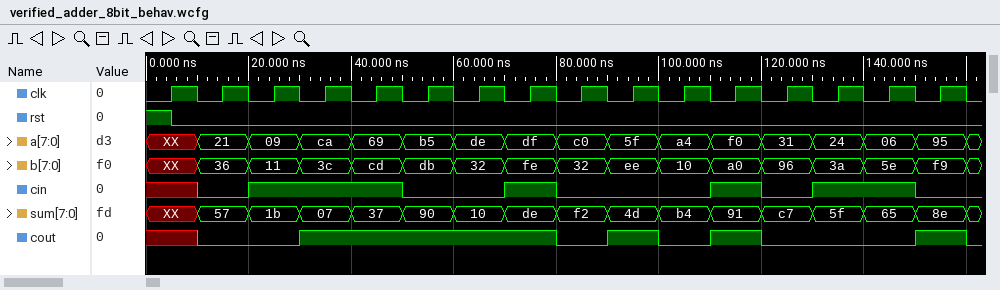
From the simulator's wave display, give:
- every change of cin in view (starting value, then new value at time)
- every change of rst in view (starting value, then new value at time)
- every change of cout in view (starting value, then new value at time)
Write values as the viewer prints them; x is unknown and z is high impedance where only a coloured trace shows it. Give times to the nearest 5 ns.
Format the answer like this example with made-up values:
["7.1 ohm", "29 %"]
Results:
["x, 0 at 10 ns, 1 at 20 ns, 0 at 50 ns, 1 at 70 ns, 0 at 80 ns, 1 at 110 ns, 0 at 120 ns, 1 at 130 ns, 0 at 150 ns", "1, 0 at 5 ns", "x, 0 at 10 ns, 1 at 30 ns, 0 at 80 ns, 1 at 90 ns, 0 at 100 ns, 1 at 110 ns, 0 at 120 ns, 1 at 150 ns, 0 at 160 ns"]
